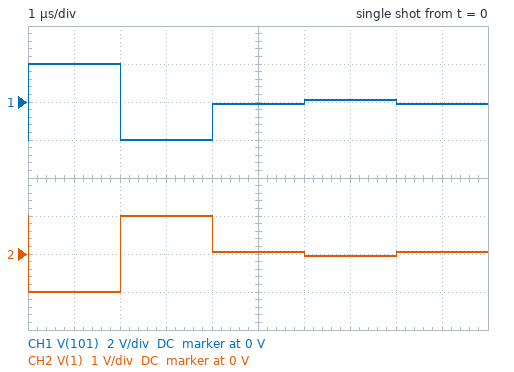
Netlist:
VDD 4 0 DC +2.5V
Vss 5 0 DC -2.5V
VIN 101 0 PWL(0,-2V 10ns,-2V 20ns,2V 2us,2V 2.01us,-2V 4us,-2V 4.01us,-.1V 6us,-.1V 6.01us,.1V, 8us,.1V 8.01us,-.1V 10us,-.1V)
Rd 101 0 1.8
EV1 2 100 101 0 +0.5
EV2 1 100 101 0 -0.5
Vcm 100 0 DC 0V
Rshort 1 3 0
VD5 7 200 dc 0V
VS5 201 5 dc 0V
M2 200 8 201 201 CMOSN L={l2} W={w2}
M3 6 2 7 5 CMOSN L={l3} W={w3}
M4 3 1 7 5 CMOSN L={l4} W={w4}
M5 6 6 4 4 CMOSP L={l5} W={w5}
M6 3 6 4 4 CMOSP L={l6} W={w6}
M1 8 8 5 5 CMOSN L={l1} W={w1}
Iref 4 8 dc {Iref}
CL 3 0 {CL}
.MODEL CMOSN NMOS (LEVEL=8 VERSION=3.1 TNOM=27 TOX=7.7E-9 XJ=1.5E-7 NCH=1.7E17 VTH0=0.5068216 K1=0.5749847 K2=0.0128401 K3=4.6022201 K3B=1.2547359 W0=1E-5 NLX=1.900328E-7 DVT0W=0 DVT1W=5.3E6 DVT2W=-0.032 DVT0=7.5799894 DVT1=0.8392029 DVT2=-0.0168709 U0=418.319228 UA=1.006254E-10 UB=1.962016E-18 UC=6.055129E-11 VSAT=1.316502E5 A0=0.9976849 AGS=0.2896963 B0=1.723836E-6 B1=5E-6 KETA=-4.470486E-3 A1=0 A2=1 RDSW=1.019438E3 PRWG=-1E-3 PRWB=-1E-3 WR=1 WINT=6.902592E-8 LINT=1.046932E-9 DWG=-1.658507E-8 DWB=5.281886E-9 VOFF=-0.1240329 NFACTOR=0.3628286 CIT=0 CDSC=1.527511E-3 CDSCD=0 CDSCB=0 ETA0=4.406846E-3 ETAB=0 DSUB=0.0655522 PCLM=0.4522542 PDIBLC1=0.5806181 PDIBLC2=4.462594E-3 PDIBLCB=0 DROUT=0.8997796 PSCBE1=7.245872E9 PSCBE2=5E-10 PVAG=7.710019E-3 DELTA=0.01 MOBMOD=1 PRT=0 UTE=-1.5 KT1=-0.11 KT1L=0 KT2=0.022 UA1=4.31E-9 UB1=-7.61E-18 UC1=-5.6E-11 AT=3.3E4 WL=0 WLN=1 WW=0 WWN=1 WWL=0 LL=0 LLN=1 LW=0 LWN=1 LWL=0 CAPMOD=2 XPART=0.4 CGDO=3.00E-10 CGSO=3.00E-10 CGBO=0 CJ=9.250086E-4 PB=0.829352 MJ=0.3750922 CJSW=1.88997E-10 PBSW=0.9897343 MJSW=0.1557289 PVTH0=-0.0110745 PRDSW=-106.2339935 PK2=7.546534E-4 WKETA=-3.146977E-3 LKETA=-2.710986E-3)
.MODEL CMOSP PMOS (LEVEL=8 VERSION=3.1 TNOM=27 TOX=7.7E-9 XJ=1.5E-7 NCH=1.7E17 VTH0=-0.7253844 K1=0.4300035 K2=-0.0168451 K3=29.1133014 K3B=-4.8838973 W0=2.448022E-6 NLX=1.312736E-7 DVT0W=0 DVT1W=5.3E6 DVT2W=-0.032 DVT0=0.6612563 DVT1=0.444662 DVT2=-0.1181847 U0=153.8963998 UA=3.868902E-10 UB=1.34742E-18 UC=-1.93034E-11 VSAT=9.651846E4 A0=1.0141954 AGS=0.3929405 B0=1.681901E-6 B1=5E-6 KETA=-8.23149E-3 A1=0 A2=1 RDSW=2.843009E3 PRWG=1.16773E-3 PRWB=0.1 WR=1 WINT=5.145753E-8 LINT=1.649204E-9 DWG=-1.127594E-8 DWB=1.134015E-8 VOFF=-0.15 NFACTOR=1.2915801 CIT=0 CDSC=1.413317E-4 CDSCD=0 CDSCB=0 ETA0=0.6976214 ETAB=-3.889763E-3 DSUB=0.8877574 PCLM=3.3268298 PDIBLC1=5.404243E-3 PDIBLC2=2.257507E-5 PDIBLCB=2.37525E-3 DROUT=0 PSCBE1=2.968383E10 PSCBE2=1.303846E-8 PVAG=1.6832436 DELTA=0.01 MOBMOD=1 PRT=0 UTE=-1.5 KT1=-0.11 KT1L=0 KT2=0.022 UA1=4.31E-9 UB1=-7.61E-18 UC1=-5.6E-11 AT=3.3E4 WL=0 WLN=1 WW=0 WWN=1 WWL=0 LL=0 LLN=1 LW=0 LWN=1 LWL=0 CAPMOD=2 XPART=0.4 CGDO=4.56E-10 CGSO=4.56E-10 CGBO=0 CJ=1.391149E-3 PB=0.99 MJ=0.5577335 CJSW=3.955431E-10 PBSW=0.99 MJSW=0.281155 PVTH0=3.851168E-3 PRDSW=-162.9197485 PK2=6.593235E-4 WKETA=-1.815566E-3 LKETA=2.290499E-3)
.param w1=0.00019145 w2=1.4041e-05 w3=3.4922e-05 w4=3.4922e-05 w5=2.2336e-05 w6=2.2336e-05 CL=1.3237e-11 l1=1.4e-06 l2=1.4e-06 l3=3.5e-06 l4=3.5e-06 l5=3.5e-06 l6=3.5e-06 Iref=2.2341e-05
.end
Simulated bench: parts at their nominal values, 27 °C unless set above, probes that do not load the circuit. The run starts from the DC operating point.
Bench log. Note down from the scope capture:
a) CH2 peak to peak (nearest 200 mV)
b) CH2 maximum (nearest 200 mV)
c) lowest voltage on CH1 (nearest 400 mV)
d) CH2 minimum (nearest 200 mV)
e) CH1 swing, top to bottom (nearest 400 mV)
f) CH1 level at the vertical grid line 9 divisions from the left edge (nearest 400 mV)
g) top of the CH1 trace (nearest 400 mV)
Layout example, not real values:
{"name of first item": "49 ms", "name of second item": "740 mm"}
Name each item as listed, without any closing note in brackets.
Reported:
{"CH2 peak to peak": "2.0 V", "CH2 maximum": "1.0 V", "lowest voltage on CH1": "-2.0 V", "CH2 minimum": "-1.0 V", "CH1 swing, top to bottom": "4.0 V", "CH1 level at the vertical grid line 9 divisions from the left edge": "0 V", "top of the CH1 trace": "2.0 V"}
